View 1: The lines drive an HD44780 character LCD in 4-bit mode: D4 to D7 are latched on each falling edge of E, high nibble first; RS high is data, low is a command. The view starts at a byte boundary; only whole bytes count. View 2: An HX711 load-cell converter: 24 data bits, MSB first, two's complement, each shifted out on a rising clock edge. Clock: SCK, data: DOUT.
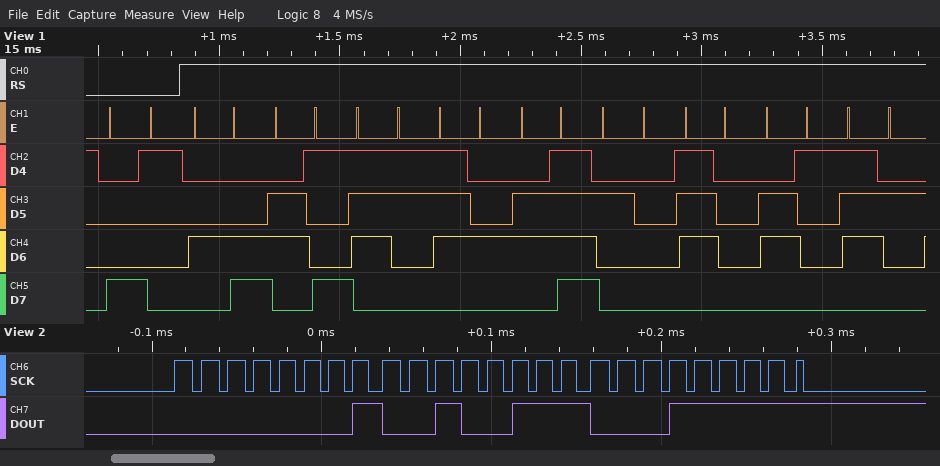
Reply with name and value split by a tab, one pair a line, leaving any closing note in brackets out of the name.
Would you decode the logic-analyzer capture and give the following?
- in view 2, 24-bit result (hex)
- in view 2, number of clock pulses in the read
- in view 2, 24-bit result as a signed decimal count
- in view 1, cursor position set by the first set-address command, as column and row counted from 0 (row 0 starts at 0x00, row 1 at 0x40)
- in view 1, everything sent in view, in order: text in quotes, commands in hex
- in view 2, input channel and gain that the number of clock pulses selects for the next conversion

in view 2, 24-bit result	0x01271F
in view 2, number of clock pulses in the read	25
in view 2, 24-bit result as a signed decimal count	75551
in view 1, cursor position set by the first set-address command, as column and row counted from 0	column 1, row 0
in view 1, everything sent in view, in order: text in quotes, commands in hex	0x81 "Listo par"
in view 2, input channel and gain that the number of clock pulses selects for the next conversion	channel A, gain 128
